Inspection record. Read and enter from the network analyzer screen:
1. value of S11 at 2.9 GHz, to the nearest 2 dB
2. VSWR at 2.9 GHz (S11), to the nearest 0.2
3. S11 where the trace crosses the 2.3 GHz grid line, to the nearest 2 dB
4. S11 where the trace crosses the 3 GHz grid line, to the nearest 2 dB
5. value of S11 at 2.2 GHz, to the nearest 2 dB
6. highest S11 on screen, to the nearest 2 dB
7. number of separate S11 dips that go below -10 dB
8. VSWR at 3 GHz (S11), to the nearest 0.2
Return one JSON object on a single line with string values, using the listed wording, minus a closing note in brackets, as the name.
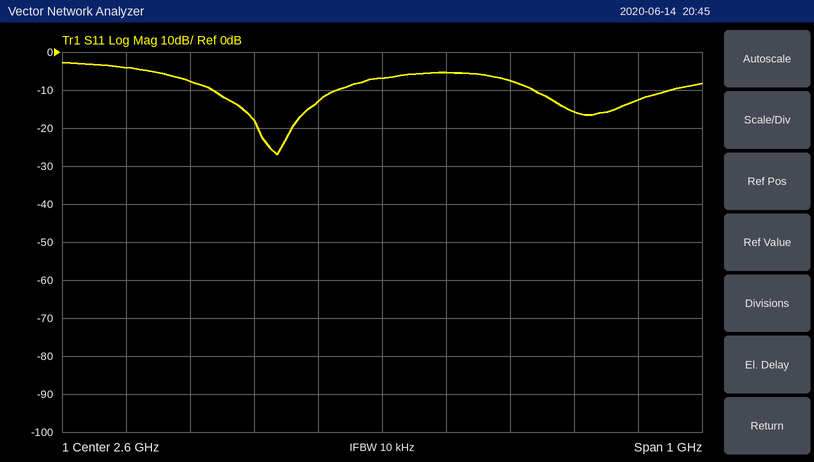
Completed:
{"value of S11 at 2.9 GHz, to the nearest 2 dB": "-16 dB", "VSWR at 2.9 GHz (S11), to the nearest 0.2": "1.4", "S11 where the trace crosses the 2.3 GHz grid line, to the nearest 2 dB": "-8 dB", "S11 where the trace crosses the 3 GHz grid line, to the nearest 2 dB": "-12 dB", "value of S11 at 2.2 GHz, to the nearest 2 dB": "-4 dB", "highest S11 on screen, to the nearest 2 dB": "-2 dB", "number of separate S11 dips that go below -10 dB": "2", "VSWR at 3 GHz (S11), to the nearest 0.2": "1.6"}
